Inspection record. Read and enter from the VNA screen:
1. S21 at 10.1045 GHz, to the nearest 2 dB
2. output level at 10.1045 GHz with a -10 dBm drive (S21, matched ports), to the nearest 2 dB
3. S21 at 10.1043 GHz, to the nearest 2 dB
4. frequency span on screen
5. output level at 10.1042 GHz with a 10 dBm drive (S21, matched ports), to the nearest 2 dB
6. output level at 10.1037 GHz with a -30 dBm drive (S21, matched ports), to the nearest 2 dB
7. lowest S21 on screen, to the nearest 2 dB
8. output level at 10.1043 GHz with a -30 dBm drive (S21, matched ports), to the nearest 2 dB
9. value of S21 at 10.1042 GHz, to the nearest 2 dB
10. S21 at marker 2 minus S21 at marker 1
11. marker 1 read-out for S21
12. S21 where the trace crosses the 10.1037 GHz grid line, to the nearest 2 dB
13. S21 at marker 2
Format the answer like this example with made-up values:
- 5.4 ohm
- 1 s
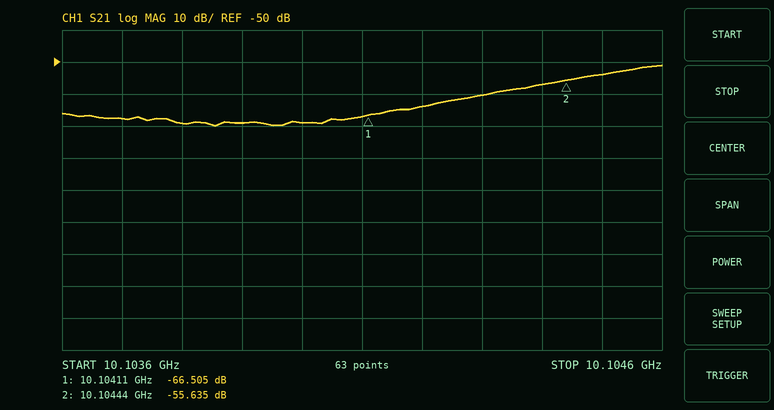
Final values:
- -54 dB
- -64 dBm
- -60 dB
- 1 MHz
- -54 dBm
- -98 dBm
- -70 dB
- -90 dBm
- -64 dB
- 10.870 dB
- -66.505 dB
- -68 dB
- -55.635 dB
